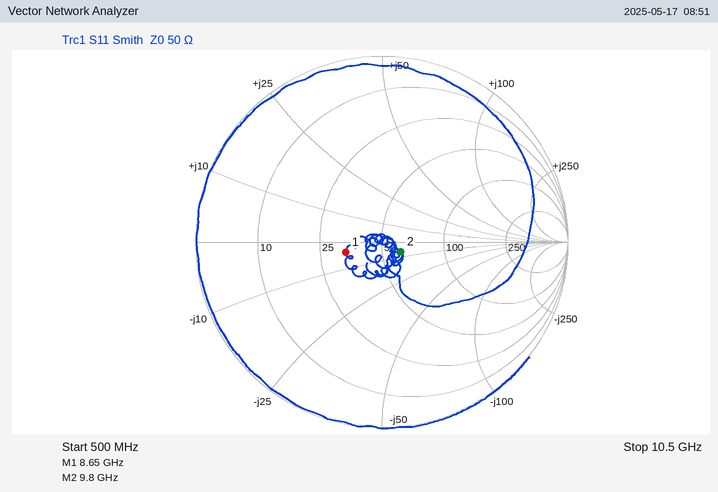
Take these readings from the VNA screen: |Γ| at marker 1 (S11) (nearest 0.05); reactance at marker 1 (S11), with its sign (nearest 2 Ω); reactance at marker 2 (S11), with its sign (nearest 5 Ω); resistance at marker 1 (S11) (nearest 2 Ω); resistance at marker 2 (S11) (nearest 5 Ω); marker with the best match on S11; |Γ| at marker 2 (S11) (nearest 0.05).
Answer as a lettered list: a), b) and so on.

a) 0.20
b) -4 Ω
c) -5 Ω
d) 34 Ω
e) 60 Ω
f) marker 2
g) 0.10
